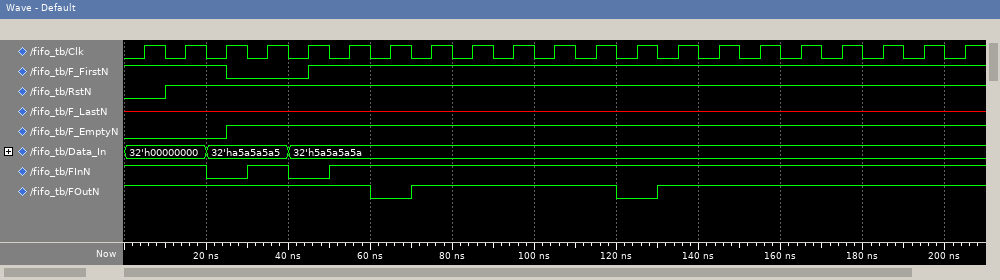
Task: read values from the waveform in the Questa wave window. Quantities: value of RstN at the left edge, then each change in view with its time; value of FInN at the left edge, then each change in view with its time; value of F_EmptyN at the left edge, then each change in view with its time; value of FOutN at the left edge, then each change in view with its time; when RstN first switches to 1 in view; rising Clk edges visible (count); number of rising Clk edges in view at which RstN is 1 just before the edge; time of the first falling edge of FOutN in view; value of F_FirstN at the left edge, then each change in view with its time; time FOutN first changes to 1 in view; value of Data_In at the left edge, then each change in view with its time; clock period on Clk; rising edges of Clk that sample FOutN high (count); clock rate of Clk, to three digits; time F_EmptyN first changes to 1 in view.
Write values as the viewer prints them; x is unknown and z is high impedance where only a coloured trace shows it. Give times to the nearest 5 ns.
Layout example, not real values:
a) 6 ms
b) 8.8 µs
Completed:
a) 0, 1 at 10 ns
b) 1, 0 at 20 ns, 1 at 30 ns, 0 at 40 ns, 1 at 50 ns
c) 0, 1 at 25 ns
d) 1, 0 at 60 ns, 1 at 70 ns, 0 at 120 ns, 1 at 130 ns
e) 10 ns
f) 21
g) 20
h) 60 ns
i) 1, 0 at 25 ns, 1 at 45 ns
j) 70 ns
k) 32'h00000000, 32'ha5a5a5a5 at 20 ns, 32'h5a5a5a5a at 40 ns
l) 10 ns
m) 19
n) 100 MHz
o) 25 ns
